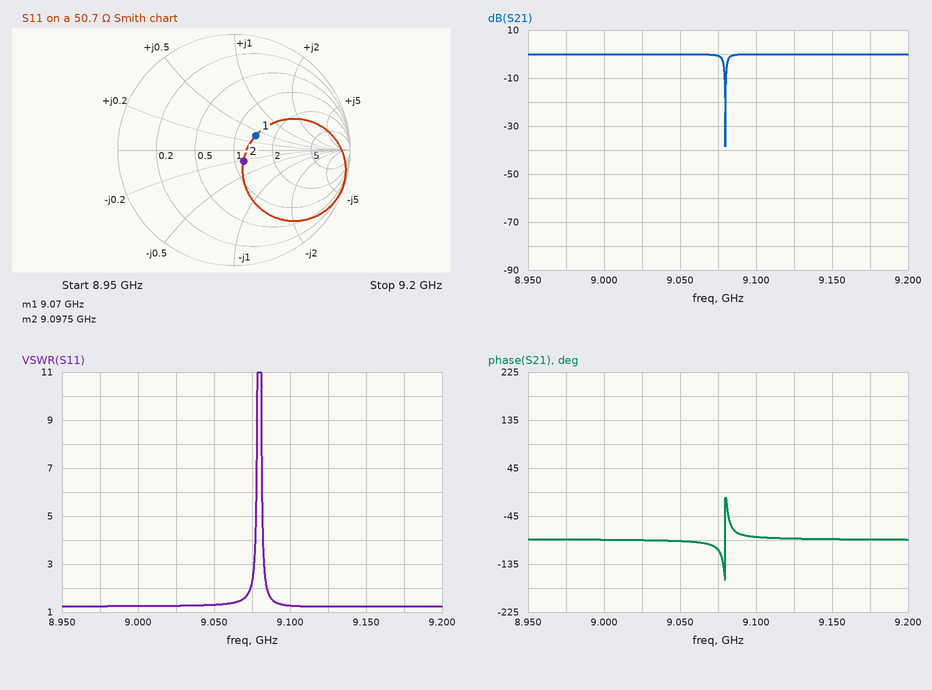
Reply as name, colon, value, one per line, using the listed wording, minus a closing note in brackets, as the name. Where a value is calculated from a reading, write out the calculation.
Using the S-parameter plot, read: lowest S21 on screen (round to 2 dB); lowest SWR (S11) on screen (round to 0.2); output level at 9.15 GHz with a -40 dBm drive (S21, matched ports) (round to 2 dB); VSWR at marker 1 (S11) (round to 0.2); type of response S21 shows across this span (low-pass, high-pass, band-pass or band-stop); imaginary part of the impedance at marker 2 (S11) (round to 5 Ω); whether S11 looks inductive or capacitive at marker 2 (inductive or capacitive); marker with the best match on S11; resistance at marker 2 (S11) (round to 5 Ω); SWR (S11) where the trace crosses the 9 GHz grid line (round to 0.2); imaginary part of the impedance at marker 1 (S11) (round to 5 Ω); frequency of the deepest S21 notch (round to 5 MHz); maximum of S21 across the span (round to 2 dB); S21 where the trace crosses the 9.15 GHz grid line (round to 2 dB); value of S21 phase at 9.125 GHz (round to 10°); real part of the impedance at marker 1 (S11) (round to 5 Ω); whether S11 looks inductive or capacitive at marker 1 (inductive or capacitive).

lowest S21 on screen: -38 dB
lowest SWR (S11) on screen: 1.2
output level at 9.15 GHz with a -40 dBm drive (S21, matched ports): -40 dBm + (0 dB) = -40 dBm
VSWR at marker 1 (S11): 1.6
type of response S21 shows across this span: band-stop
imaginary part of the impedance at marker 2 (S11): -10 Ω
whether S11 looks inductive or capacitive at marker 2: capacitive
marker with the best match on S11: marker 2
resistance at marker 2 (S11): 60 Ω
SWR (S11) where the trace crosses the 9 GHz grid line: 1.2
imaginary part of the impedance at marker 1 (S11): +20 Ω
frequency of the deepest S21 notch: 9.080 GHz
maximum of S21 across the span: 0 dB
S21 where the trace crosses the 9.15 GHz grid line: 0 dB
value of S21 phase at 9.125 GHz: -90°
real part of the impedance at marker 1 (S11): 70 Ω
whether S11 looks inductive or capacitive at marker 1: inductive
